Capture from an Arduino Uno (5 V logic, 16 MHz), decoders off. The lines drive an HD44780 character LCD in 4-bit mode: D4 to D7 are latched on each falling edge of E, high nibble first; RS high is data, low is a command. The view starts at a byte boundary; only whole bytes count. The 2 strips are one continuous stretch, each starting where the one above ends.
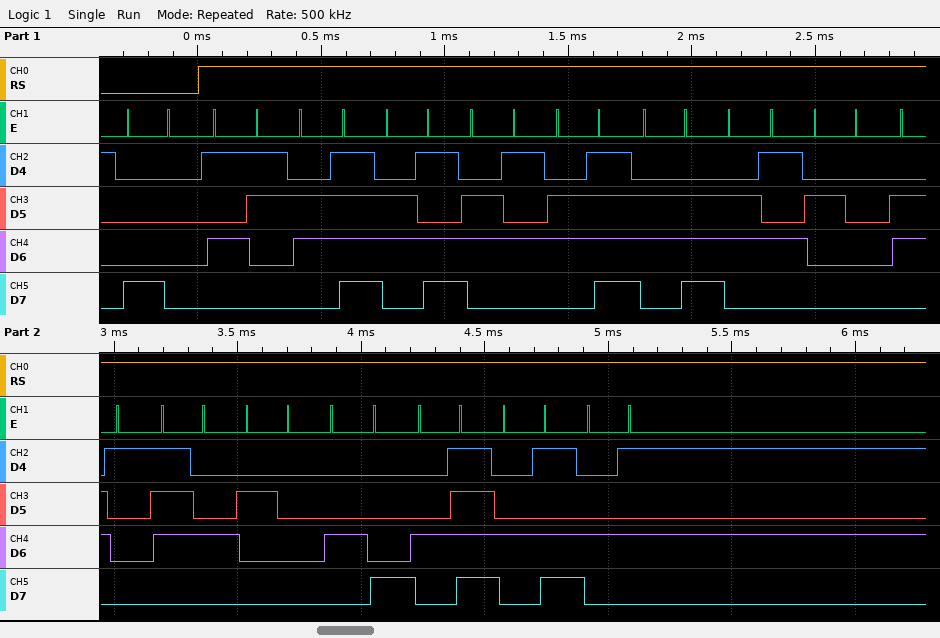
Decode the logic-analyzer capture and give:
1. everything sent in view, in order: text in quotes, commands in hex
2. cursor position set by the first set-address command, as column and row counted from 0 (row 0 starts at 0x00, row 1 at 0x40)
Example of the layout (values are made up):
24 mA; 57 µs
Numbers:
0x80 "Someone at HOME"; column 0, row 0
